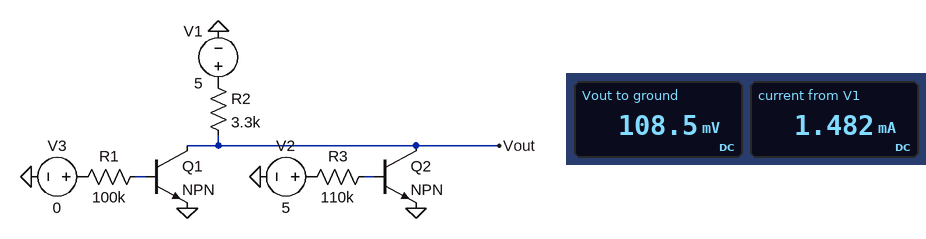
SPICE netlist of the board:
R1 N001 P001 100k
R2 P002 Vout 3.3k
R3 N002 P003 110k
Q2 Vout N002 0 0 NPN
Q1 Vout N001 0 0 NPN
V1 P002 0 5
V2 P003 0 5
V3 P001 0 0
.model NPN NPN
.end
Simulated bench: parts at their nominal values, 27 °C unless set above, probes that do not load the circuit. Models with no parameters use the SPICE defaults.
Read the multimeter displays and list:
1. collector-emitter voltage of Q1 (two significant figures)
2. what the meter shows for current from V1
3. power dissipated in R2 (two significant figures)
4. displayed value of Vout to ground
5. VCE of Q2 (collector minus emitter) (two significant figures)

110 mV
1.482 mA
7.3 mW
108.5 mV
110 mV
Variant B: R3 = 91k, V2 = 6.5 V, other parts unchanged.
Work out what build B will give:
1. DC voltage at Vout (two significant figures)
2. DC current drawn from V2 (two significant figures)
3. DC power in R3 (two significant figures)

91 mV
63 µA
360 µW
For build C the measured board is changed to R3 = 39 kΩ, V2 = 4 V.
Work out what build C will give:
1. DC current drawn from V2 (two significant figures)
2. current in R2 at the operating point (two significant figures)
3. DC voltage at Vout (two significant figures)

82 µA
1.5 mA
83 mV
